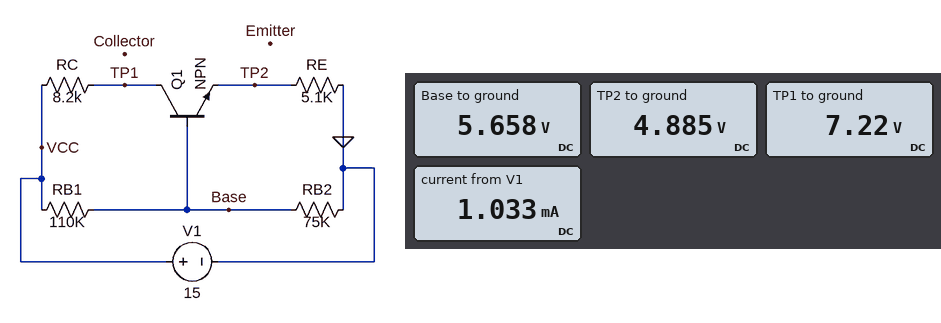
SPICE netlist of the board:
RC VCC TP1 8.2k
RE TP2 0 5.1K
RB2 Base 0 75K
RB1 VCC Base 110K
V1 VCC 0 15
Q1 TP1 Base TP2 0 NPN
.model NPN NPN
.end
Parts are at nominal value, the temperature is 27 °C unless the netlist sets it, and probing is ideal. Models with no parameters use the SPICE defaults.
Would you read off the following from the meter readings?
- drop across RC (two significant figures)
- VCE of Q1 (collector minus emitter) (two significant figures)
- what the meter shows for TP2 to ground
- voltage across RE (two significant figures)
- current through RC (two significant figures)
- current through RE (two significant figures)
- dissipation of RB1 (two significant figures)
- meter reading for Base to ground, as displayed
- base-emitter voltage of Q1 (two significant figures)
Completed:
7.8 V
2.3 V
4.885 V
4.9 V
950 µA
960 µA
790 µW
5.658 V
770 mV
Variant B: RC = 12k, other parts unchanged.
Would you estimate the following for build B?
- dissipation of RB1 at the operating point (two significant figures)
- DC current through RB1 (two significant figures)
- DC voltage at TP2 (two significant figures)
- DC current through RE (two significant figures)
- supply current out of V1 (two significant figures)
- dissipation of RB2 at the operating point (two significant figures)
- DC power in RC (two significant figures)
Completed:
860 µW
88 µA
4.5 V
880 µA
950 µA
370 µW
9.0 mW
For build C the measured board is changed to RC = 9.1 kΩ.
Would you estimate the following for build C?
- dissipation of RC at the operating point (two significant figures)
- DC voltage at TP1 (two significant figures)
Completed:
8.2 mW
6.4 V
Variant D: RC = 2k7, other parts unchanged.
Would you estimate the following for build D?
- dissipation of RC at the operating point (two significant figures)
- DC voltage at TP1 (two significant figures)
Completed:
2.4 mW
12 V
